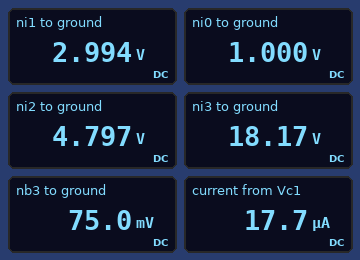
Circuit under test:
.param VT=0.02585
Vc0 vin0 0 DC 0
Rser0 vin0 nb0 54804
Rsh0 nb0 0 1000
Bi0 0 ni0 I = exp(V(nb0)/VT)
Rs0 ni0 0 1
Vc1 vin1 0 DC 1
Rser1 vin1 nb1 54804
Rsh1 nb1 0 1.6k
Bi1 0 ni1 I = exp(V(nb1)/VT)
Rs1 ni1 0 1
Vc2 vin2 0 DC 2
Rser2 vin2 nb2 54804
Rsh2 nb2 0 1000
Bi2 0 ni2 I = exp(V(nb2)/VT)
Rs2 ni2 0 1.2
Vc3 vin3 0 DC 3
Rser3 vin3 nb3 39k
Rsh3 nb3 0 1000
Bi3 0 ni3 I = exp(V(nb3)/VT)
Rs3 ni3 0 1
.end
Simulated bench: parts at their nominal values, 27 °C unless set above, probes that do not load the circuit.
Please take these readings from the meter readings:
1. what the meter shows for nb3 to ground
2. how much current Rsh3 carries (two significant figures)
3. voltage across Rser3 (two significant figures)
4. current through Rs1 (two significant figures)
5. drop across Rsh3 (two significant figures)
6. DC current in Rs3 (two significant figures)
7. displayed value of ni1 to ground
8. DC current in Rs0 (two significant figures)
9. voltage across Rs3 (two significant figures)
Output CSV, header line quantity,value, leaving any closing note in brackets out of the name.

quantity,value
what the meter shows for nb3 to ground,75.0 mV
how much current Rsh3 carries,75 µA
voltage across Rser3,2.9 V
current through Rs1,3.0 A
drop across Rsh3,75 mV
DC current in Rs3,18 A
displayed value of ni1 to ground,2.994 V
DC current in Rs0,1.0 A
voltage across Rs3,18 V
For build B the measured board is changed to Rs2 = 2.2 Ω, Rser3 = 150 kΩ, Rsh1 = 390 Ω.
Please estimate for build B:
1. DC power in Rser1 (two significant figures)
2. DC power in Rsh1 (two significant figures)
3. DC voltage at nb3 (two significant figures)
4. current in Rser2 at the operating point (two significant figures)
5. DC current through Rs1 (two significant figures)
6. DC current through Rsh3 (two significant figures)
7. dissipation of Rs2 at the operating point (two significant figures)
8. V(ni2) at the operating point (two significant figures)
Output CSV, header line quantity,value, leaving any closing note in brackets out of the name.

quantity,value
DC power in Rser1,18 µW
DC power in Rsh1,130 nW
DC voltage at nb3,20 mV
current in Rser2 at the operating point,36 µA
DC current through Rs1,1.3 A
DC current through Rsh3,20 µA
dissipation of Rs2 at the operating point,35 W
V(ni2) at the operating point,8.8 V
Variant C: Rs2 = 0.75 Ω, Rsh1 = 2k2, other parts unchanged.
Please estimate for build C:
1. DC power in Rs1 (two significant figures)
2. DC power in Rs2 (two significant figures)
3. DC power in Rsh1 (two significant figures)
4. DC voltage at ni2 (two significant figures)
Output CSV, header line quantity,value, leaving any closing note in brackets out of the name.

quantity,value
DC power in Rs1,20 W
DC power in Rs2,12 W
DC power in Rsh1,680 nW
DC voltage at ni2,3.0 V
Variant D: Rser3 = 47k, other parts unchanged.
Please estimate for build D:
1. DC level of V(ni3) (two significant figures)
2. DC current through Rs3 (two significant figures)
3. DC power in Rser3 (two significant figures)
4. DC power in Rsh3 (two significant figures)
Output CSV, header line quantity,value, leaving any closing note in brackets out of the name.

quantity,value
DC level of V(ni3),11 V
DC current through Rs3,11 A
DC power in Rser3,180 µW
DC power in Rsh3,3.9 µW
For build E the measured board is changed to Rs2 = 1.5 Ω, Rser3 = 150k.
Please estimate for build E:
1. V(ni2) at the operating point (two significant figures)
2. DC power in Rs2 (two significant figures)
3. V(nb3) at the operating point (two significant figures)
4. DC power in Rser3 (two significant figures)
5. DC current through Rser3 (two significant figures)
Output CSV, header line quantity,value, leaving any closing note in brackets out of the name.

quantity,value
V(ni2) at the operating point,6.0 V
DC power in Rs2,24 W
V(nb3) at the operating point,20 mV
DC power in Rser3,59 µW
DC current through Rser3,20 µA
